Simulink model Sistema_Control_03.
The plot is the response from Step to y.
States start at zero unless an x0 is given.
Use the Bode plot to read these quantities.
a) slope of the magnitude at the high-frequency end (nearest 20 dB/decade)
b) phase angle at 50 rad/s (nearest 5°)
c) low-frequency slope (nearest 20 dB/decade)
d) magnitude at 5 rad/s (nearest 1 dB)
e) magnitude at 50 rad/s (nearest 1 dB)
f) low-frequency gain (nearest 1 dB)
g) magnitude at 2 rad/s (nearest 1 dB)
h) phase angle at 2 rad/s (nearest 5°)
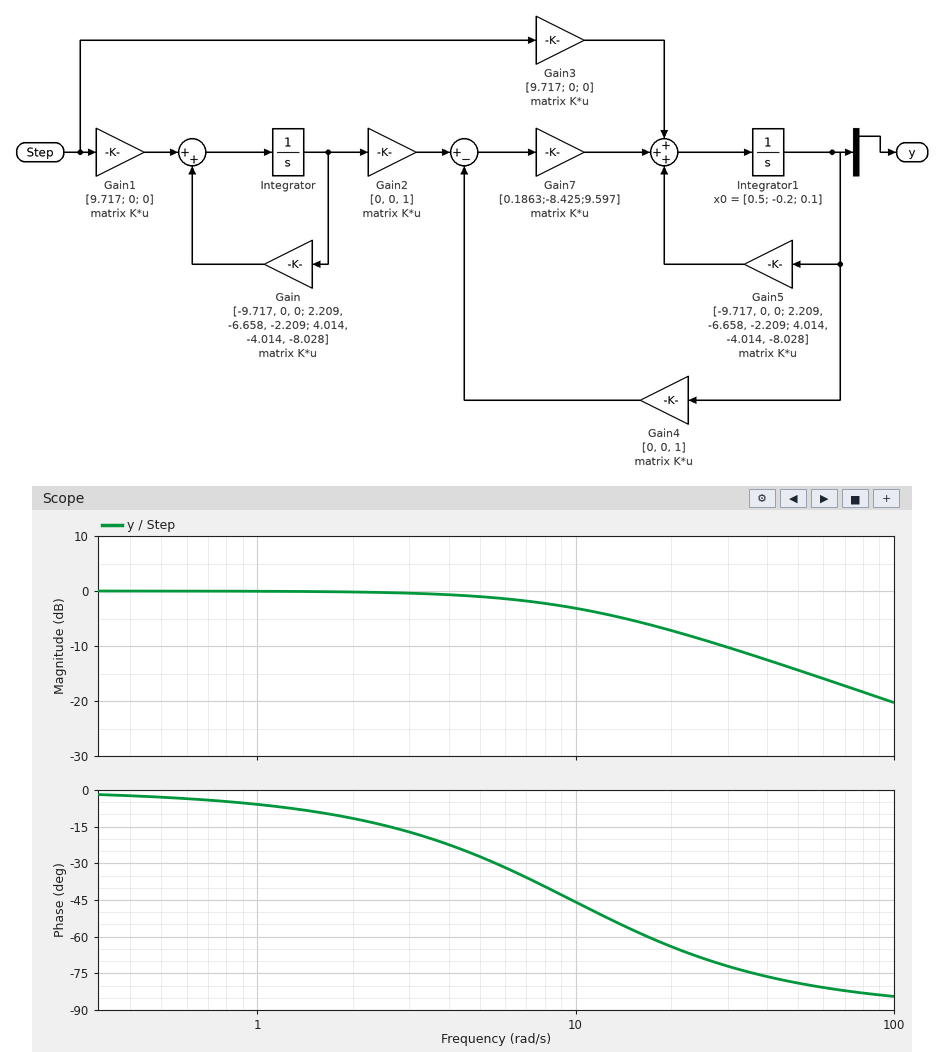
-20 dB/decade
-80°
0 dB/decade
-1 dB
-14 dB
0 dB
0 dB
-10°
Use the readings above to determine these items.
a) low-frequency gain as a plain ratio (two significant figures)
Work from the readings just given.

1.0
